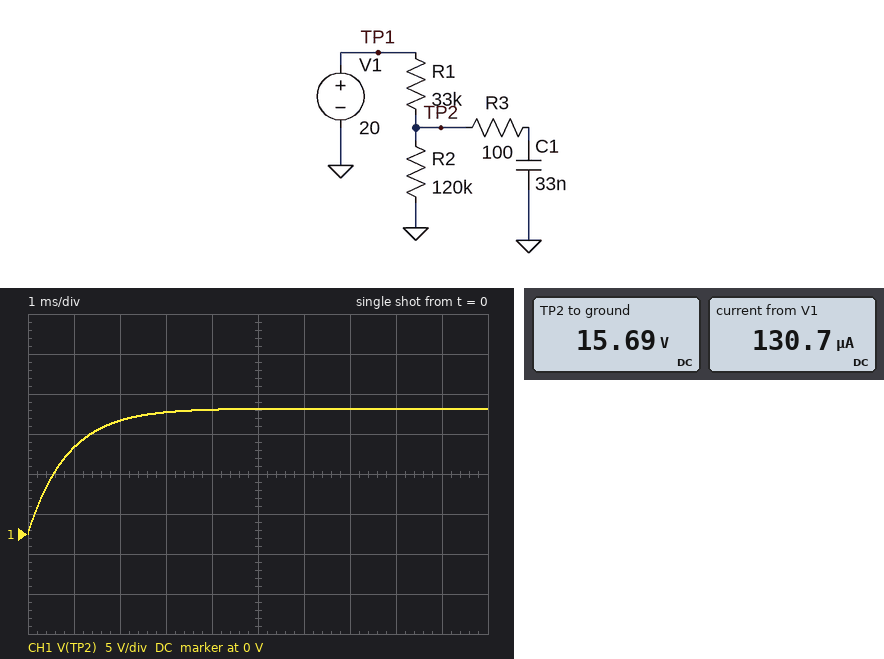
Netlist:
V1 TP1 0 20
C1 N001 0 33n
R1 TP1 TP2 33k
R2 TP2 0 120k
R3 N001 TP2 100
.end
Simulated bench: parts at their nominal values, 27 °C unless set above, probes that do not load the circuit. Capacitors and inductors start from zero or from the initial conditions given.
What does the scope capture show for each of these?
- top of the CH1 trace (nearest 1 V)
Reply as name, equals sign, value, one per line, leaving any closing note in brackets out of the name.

top of the CH1 trace = 16 V
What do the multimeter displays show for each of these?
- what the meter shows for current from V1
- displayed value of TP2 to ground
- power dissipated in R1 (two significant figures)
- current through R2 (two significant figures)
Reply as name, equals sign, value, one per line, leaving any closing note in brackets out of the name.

what the meter shows for current from V1 = 130.7 µA
displayed value of TP2 to ground = 15.69 V
power dissipated in R1 = 560 µW
current through R2 = 130 µA
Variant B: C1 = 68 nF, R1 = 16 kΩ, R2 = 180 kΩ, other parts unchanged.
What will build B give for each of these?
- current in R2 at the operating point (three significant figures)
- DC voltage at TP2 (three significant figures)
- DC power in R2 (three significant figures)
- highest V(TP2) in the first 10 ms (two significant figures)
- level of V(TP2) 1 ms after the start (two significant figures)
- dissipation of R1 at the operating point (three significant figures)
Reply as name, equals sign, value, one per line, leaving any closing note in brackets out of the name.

current in R2 at the operating point = 102 µA
DC voltage at TP2 = 18.4 V
DC power in R2 = 1.87 mW
highest V(TP2) in the first 10 ms = 18 V
level of V(TP2) 1 ms after the start = 12 V
dissipation of R1 at the operating point = 167 µW
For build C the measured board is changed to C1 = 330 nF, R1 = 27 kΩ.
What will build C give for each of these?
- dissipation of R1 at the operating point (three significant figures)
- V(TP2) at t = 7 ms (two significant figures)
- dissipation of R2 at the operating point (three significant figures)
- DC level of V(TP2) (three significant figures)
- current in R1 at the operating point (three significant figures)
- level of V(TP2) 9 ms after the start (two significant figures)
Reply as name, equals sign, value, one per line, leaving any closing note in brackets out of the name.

dissipation of R1 at the operating point = 500 µW
V(TP2) at t = 7 ms = 10 V
dissipation of R2 at the operating point = 2.22 mW
DC level of V(TP2) = 16.3 V
current in R1 at the operating point = 136 µA
level of V(TP2) 9 ms after the start = 12 V
